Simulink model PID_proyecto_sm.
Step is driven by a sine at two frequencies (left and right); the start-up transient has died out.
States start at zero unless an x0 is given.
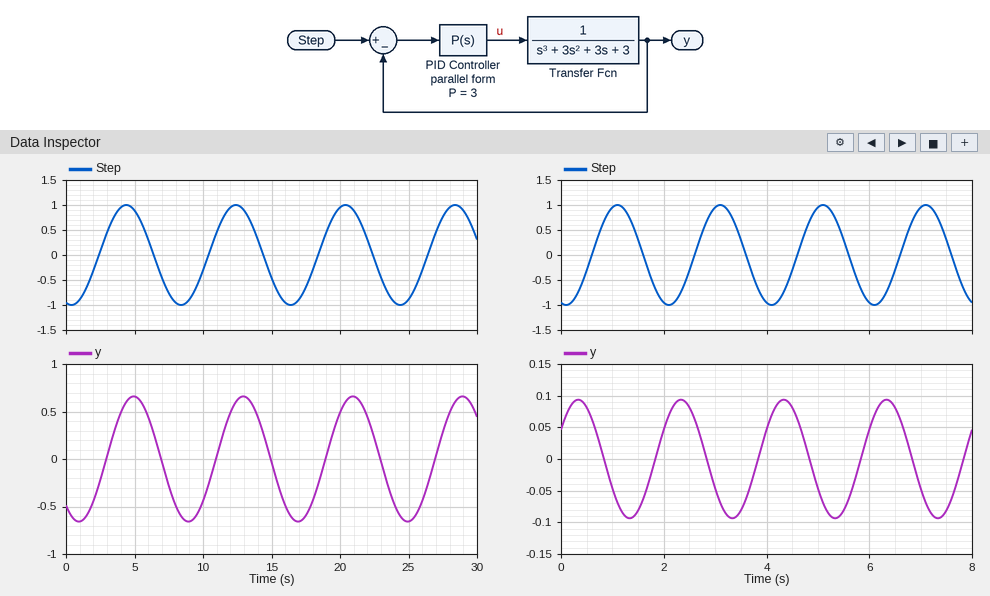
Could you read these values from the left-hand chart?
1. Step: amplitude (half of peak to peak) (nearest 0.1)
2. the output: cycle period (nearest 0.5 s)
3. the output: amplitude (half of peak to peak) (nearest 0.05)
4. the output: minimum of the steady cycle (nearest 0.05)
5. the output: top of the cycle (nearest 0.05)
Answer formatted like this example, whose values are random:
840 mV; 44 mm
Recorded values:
1.0; 8.0 s; 0.65; -0.65; 0.65
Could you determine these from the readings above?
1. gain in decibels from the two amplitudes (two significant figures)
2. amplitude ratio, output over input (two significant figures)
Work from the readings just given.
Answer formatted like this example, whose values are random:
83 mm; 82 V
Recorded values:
-3.7 dB; 0.65
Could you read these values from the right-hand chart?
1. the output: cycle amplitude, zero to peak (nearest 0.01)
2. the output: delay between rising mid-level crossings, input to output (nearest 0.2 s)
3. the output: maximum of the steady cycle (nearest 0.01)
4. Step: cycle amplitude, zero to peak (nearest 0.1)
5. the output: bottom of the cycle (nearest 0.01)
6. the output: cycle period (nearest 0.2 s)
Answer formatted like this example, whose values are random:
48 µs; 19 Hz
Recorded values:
0.09; 1.2 s; 0.09; 1.0; -0.09; 2.0 s
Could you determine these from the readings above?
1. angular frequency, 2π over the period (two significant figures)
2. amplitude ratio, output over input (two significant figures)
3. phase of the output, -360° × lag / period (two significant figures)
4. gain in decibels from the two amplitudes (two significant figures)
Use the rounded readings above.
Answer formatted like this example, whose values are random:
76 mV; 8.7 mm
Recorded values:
3.1 rad/s; 0.090; -220°; -21 dB
